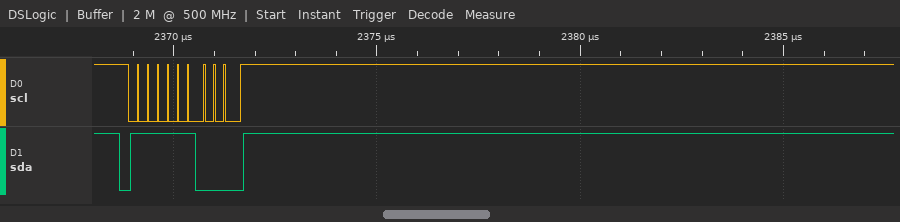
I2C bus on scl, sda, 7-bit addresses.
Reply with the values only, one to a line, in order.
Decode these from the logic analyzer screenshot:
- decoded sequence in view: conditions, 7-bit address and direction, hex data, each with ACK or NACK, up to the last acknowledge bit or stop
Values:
start, address 7E write ACK, stop
